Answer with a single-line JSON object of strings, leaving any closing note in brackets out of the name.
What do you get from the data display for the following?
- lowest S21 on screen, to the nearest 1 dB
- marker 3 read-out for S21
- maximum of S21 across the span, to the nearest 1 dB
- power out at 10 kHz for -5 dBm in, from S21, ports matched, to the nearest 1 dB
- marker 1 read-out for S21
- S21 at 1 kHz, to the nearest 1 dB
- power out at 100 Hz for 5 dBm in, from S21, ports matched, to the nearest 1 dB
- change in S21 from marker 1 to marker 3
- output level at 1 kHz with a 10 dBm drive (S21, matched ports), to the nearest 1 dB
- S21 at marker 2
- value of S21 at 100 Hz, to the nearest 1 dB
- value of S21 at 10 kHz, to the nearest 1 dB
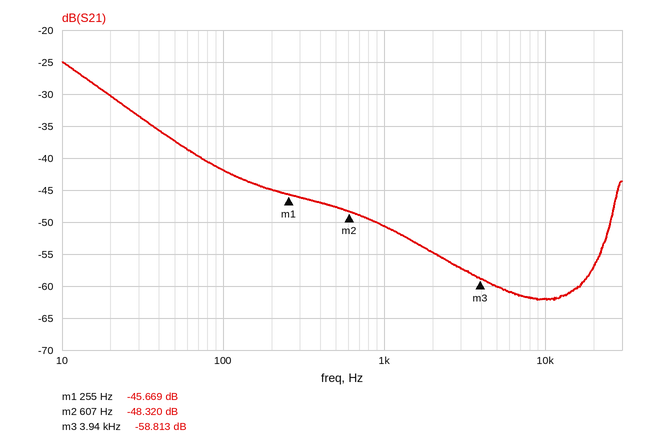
{"lowest S21 on screen, to the nearest 1 dB": "-62 dB", "marker 3 read-out for S21": "-58.813 dB", "maximum of S21 across the span, to the nearest 1 dB": "-25 dB", "power out at 10 kHz for -5 dBm in, from S21, ports matched, to the nearest 1 dB": "-67 dBm", "marker 1 read-out for S21": "-45.669 dB", "S21 at 1 kHz, to the nearest 1 dB": "-51 dB", "power out at 100 Hz for 5 dBm in, from S21, ports matched, to the nearest 1 dB": "-37 dBm", "change in S21 from marker 1 to marker 3": "-13.144 dB", "output level at 1 kHz with a 10 dBm drive (S21, matched ports), to the nearest 1 dB": "-41 dBm", "S21 at marker 2": "-48.320 dB", "value of S21 at 100 Hz, to the nearest 1 dB": "-42 dB", "value of S21 at 10 kHz, to the nearest 1 dB": "-62 dB"}
